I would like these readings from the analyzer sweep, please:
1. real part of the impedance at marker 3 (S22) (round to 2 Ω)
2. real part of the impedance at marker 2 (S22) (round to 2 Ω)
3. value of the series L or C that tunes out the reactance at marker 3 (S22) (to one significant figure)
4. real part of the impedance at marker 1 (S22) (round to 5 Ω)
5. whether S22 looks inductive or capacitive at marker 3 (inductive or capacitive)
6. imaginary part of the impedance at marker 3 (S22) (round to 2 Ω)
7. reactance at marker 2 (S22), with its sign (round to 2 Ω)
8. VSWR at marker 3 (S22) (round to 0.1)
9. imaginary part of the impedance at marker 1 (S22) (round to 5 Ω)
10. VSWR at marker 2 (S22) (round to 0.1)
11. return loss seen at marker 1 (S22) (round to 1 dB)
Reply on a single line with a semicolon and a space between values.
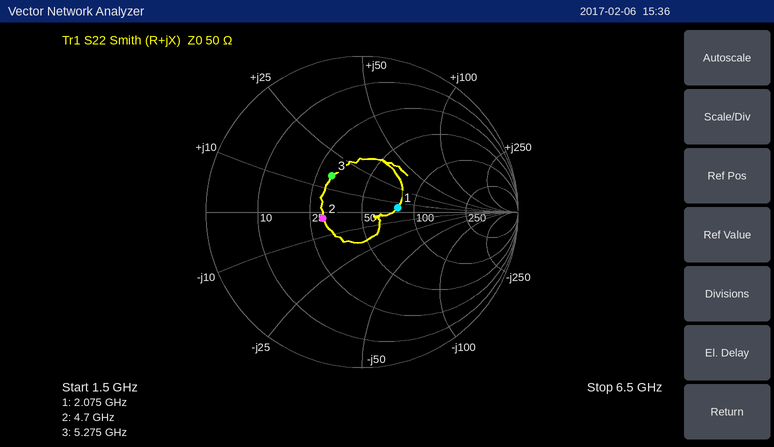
30 Ω; 30 Ω; 2 pF; 80 Ω; inductive; +16 Ω; -2 Ω; 1.9; +5 Ω; 1.7; 13 dB
